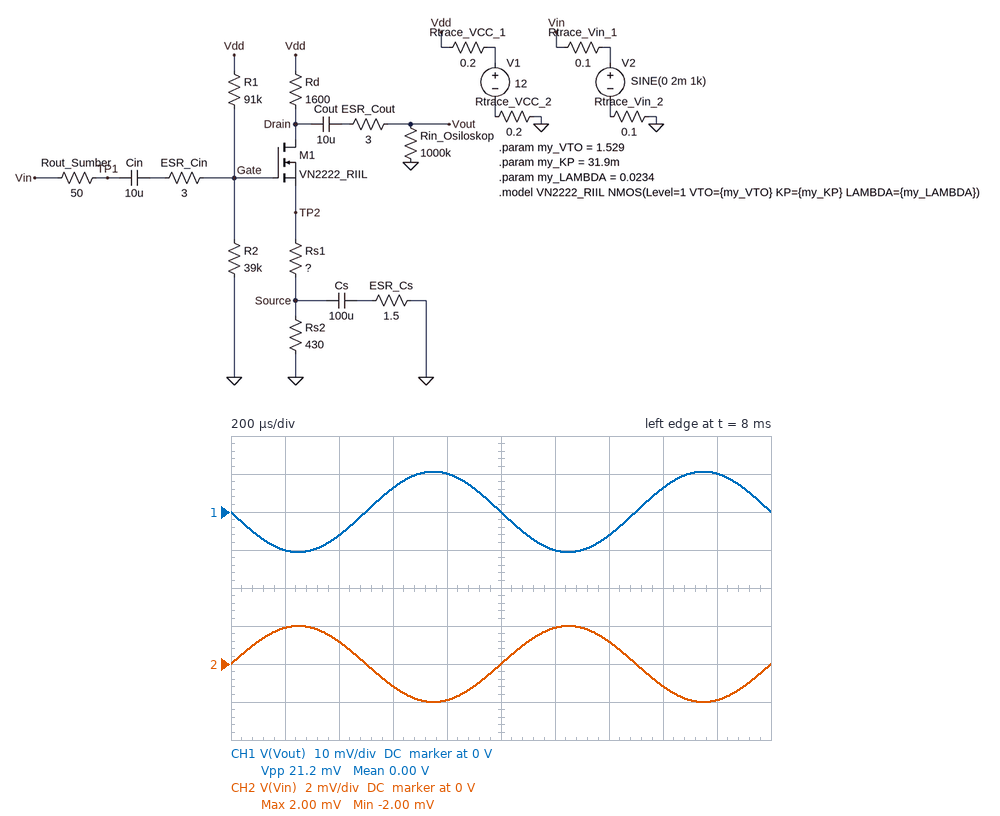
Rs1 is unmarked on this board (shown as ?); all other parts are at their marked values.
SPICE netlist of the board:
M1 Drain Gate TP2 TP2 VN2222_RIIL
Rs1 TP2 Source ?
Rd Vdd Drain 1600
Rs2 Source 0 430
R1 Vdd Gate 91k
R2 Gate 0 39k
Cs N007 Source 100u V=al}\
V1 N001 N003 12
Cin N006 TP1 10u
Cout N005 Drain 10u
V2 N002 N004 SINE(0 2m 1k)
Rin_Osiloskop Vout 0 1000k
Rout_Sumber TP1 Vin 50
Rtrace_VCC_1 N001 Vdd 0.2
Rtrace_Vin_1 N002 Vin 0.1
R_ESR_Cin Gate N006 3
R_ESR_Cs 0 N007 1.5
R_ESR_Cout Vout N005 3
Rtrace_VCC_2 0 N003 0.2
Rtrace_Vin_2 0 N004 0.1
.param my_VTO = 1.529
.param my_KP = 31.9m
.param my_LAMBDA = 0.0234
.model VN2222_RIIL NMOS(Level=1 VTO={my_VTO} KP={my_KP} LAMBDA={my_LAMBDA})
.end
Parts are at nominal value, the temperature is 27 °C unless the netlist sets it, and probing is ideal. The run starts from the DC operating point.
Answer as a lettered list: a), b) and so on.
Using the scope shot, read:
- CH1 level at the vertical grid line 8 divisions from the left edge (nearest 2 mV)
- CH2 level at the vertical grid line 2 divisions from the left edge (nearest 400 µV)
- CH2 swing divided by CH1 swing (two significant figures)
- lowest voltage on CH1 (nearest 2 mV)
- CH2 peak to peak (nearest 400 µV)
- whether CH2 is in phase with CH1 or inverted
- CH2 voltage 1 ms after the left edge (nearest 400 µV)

a) 6 mV
b) 1.2 mV
c) 0.19
d) -10 mV
e) 4.0 mV
f) inverted
g) 0 V
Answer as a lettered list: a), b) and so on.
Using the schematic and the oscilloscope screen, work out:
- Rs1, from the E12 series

a) 220 Ω
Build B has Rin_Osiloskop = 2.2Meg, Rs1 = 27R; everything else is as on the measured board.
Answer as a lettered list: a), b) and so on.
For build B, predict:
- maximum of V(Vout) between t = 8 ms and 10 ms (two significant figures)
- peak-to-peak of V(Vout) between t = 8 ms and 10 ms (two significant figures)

a) 32 mV
b) 64 mV
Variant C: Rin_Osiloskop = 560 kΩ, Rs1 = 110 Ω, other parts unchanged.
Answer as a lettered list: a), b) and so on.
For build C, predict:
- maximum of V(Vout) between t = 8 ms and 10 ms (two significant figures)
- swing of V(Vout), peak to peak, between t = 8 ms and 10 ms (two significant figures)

a) 17 mV
b) 34 mV
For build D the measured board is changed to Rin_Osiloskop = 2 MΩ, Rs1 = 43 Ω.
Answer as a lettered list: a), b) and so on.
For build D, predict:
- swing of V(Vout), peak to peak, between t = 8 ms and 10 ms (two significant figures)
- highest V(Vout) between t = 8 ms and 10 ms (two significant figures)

a) 55 mV
b) 28 mV
